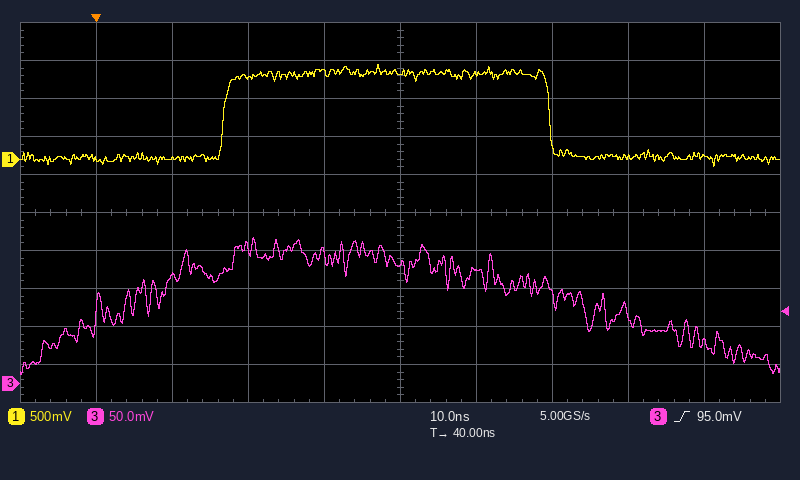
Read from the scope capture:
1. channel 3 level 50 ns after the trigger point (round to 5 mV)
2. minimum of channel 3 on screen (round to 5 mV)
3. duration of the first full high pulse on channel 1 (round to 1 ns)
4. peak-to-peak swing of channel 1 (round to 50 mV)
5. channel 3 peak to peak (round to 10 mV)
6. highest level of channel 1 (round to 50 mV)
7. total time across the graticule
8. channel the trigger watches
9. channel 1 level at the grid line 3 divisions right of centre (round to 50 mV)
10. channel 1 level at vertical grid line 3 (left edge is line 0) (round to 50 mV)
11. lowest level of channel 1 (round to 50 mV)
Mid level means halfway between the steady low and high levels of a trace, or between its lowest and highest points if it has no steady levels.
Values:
150 mV
10 mV
43 ns
1.35 V
180 mV
1.25 V
100 ns
channel 3
50 mV
1.10 V
-100 mV
